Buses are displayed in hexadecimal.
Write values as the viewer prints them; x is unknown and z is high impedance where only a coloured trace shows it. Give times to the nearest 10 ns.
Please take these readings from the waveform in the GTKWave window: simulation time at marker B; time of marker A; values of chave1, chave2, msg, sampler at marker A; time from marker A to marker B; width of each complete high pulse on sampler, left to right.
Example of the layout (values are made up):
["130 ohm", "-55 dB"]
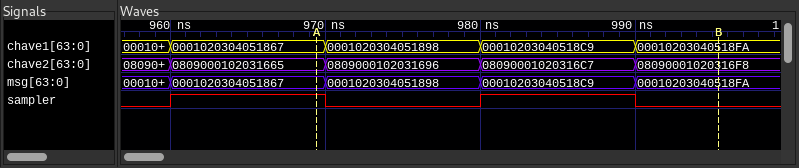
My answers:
["1000 ns", "970 ns", "chave1=0001020304051867, chave2=0809000102031665, msg=0001020304051867, sampler=1", "30 ns", "10 ns, 10 ns"]
